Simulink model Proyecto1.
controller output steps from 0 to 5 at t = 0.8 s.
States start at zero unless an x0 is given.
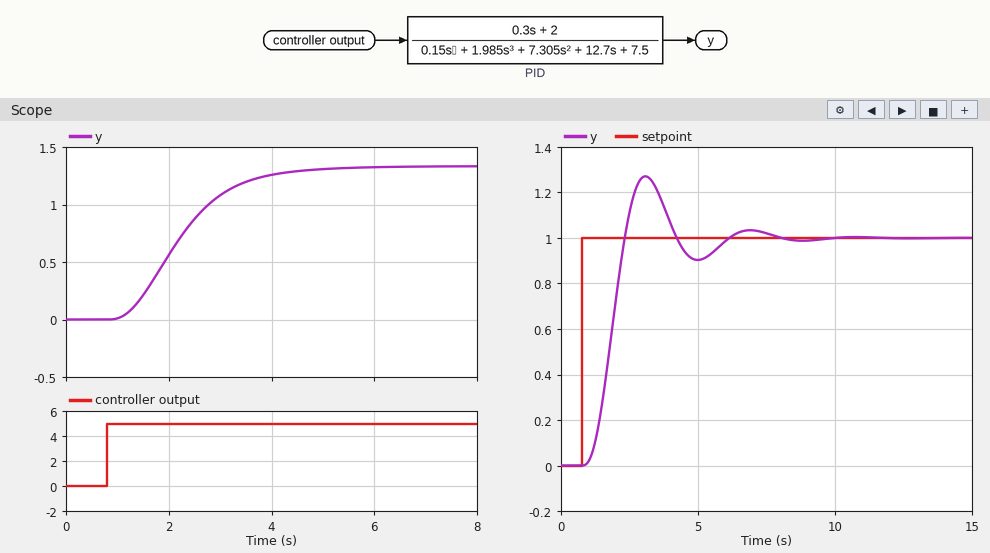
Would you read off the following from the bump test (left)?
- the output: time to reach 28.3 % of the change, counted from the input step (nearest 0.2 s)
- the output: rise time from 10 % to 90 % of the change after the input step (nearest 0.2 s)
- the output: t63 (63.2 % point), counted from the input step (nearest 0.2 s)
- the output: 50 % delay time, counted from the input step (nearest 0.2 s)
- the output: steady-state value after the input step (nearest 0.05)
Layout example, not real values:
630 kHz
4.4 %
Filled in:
1.0 s
2.2 s
1.6 s
1.4 s
1.35
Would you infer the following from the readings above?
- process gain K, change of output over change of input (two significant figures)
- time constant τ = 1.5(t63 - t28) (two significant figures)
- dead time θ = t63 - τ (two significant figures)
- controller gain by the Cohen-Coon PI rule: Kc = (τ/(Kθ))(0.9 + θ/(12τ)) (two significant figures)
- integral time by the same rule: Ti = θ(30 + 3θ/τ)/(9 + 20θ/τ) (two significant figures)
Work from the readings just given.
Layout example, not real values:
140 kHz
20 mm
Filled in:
0.27
0.90 s
0.70 s
4.6
0.92 s
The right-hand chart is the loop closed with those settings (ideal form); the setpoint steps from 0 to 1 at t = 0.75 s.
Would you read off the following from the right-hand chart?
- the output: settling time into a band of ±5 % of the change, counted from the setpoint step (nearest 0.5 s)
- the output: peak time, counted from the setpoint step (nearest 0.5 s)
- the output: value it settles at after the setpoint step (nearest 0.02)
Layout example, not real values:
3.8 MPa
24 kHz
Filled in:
5.0 s
2.5 s
1.00
